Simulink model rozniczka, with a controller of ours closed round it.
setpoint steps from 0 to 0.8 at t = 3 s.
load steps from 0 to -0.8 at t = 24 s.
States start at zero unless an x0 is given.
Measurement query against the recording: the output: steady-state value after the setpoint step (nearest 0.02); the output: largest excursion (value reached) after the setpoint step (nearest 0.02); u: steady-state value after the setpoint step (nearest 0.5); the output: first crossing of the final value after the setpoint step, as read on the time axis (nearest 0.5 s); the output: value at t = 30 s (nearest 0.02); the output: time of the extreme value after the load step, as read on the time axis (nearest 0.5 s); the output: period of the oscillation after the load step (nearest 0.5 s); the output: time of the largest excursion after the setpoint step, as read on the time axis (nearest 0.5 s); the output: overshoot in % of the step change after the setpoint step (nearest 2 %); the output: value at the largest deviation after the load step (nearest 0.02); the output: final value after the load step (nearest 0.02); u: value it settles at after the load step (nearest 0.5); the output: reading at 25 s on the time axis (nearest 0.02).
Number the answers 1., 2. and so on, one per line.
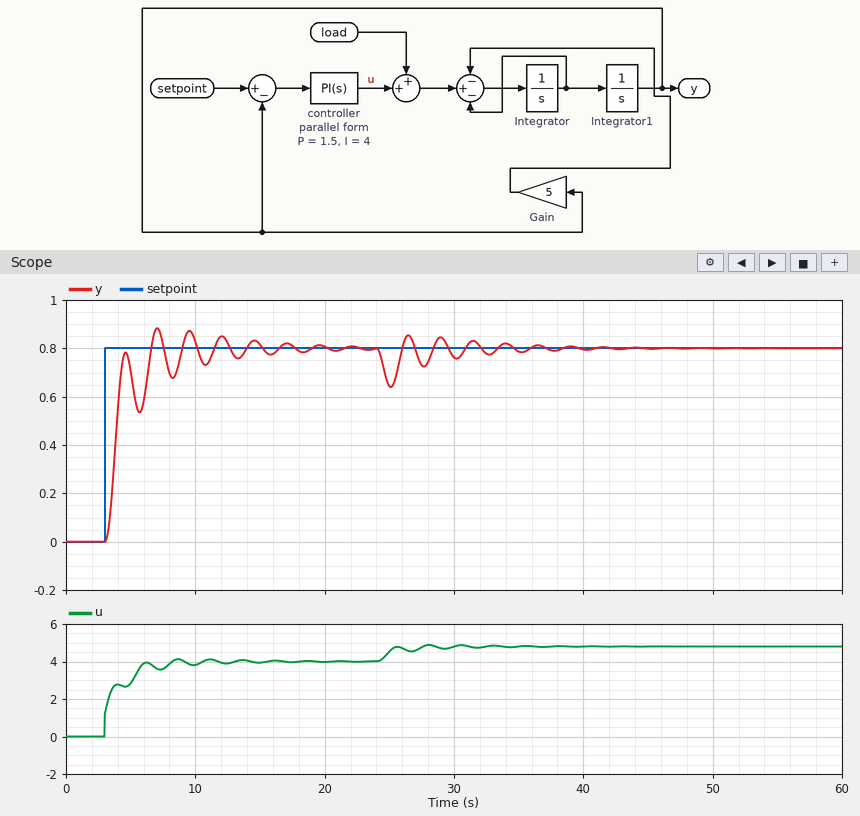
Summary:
1. 0.80
2. 0.88
3. 4.0
4. 6.5 s
5. 0.76
6. 25.0 s
7. 2.5 s
8. 7.0 s
9. 10 %
10. 0.64
11. 0.80
12. 5.0
13. 0.64
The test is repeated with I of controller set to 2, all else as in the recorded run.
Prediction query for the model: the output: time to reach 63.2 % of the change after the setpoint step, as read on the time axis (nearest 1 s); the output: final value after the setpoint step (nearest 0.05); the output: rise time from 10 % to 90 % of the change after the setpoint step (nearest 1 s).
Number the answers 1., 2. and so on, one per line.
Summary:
1. 4 s
2. 0.80
3. 6 s
